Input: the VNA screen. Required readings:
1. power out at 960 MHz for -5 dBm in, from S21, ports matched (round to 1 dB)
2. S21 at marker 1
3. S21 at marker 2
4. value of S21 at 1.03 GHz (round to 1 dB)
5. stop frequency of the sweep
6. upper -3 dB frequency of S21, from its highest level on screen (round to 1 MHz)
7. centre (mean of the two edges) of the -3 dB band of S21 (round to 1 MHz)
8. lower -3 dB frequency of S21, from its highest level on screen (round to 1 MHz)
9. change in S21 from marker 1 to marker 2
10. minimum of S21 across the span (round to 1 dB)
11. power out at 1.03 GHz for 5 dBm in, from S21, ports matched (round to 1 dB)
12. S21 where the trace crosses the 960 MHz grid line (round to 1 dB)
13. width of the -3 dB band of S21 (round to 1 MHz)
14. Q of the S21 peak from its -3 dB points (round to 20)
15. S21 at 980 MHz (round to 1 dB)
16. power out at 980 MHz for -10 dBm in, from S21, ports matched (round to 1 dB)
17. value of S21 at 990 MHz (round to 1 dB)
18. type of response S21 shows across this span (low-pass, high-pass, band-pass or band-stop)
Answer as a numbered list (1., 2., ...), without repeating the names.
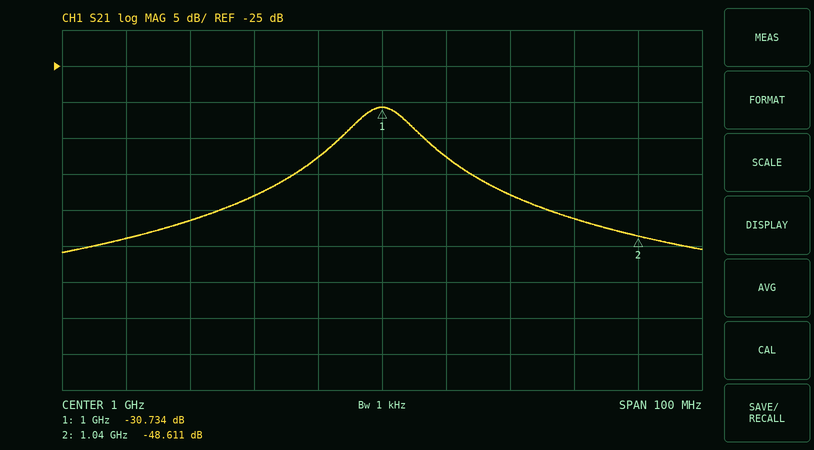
1. -54 dBm
2. -30.734 dB
3. -48.611 dB
4. -46 dB
5. 1.05 GHz
6. 1.005 GHz
7. 1.000 GHz
8. 995 MHz
9. -17.877 dB
10. -51 dB
11. -41 dBm
12. -49 dB
13. 10 MHz
14. 100
15. -43 dB
16. -53 dBm
17. -38 dB
18. band-pass
